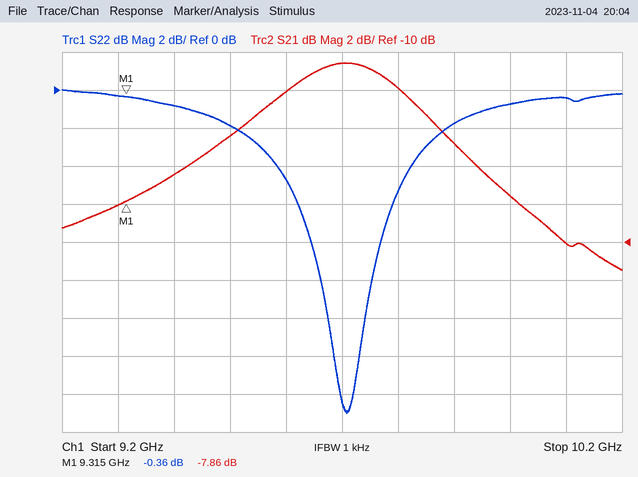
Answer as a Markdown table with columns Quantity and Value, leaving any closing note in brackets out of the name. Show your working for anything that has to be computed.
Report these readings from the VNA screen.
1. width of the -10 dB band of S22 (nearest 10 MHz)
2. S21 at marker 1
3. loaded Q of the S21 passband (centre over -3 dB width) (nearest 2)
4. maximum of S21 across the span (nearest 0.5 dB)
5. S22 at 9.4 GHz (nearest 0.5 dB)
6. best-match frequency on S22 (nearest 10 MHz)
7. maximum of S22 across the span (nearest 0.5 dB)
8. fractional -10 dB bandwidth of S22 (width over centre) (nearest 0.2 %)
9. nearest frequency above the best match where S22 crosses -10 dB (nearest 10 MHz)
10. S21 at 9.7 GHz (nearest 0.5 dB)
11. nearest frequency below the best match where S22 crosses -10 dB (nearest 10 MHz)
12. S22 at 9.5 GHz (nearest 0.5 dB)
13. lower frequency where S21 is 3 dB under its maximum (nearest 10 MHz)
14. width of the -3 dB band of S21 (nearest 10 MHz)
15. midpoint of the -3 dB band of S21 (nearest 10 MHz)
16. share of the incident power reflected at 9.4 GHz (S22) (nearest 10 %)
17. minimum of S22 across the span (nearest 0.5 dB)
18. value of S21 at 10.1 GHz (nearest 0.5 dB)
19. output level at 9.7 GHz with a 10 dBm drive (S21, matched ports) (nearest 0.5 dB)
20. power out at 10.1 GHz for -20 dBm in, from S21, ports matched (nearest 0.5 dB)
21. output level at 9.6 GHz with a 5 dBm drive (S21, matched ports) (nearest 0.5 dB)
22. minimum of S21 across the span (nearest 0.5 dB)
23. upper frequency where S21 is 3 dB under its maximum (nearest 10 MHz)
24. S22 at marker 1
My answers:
| Quantity | Value |
|---|---|
| width of the -10 dB band of S22 | 9.75 GHz − 9.66 GHz = 90 MHz |
| S21 at marker 1 | -7.86 dB |
| loaded Q of the S21 passband (centre over -3 dB width) | 9.7 GHz / 320 MHz ≈ 30 |
| maximum of S21 across the span | -0.5 dB |
| S22 at 9.4 GHz | -1.0 dB |
| best-match frequency on S22 | 9.71 GHz |
| maximum of S22 across the span | 0.0 dB |
| fractional -10 dB bandwidth of S22 (width over centre) | 90 MHz / 9.705 GHz ≈ 0.927 %, so 1.0 % to the nearest 0.2 % |
| nearest frequency above the best match where S22 crosses -10 dB | 9.75 GHz |
| S21 at 9.7 GHz | -0.5 dB |
| nearest frequency below the best match where S22 crosses -10 dB | 9.66 GHz |
| S22 at 9.5 GHz | -2.0 dB |
| lower frequency where S21 is 3 dB under its maximum | 9.54 GHz |
| width of the -3 dB band of S21 | 9.86 GHz − 9.54 GHz = 320 MHz |
| midpoint of the -3 dB band of S21 | 9.70 GHz |
| share of the incident power reflected at 9.4 GHz (S22) | 10^(-1/10) ≈ 79.4 %, so 80 % to the nearest 10 % |
| minimum of S22 across the span | -17.0 dB |
| value of S21 at 10.1 GHz | -10.0 dB |
| output level at 9.7 GHz with a 10 dBm drive (S21, matched ports) | 10 dBm + (-0.5 dB) = 9.5 dBm |
| power out at 10.1 GHz for -20 dBm in, from S21, ports matched | -20 dBm + (-10.0 dB) = -30.0 dBm |
| output level at 9.6 GHz with a 5 dBm drive (S21, matched ports) | 5 dBm + (-2.0 dB) = 3.0 dBm |
| minimum of S21 across the span | -11.5 dB |
| upper frequency where S21 is 3 dB under its maximum | 9.86 GHz |
| S22 at marker 1 | -0.36 dB |
